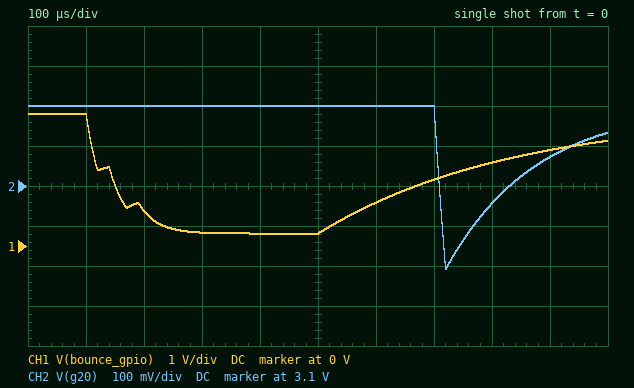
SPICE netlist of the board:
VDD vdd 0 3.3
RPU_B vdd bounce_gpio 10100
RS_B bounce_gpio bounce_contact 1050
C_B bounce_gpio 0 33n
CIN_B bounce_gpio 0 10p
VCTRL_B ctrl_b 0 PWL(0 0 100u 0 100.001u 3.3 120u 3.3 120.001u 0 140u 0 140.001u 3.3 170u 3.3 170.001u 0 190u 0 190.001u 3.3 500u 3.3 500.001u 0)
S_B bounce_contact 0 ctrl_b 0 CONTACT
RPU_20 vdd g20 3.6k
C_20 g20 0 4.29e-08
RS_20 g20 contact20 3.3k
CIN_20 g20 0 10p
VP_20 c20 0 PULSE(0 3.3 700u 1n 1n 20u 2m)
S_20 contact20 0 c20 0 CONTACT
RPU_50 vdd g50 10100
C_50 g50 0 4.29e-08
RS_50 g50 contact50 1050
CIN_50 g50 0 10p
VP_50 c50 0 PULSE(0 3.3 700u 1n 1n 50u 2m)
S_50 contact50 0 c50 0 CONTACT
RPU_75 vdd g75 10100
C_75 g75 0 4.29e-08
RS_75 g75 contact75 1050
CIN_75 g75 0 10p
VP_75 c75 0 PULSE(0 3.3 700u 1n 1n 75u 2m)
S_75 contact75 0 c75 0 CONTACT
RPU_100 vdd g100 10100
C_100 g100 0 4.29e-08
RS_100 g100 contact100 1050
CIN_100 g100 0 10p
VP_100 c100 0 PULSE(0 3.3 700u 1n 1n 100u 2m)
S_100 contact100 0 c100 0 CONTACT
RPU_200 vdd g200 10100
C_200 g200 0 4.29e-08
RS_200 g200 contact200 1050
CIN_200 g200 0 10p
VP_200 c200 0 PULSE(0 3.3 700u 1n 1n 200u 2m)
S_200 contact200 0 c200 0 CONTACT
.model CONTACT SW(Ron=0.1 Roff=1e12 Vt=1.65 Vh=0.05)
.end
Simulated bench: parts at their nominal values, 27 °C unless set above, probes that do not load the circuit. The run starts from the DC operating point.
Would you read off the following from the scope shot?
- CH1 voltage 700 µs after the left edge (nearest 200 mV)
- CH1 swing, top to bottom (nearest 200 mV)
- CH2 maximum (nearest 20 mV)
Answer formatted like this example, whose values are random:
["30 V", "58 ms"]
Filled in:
["1.6 V", "3.0 V", "3.30 V"]
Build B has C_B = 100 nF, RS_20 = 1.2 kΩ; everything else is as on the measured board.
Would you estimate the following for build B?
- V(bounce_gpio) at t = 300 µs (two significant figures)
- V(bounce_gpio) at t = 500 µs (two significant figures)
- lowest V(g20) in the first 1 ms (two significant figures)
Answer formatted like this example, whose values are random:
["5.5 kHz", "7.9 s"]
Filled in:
["880 mV", "380 mV", "2.3 V"]
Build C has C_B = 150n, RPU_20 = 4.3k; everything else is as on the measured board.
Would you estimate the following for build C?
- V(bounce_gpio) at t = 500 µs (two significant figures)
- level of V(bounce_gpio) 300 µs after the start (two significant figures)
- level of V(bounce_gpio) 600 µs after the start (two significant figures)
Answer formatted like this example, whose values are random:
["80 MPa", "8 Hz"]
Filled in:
["550 mV", "1.3 V", "730 mV"]
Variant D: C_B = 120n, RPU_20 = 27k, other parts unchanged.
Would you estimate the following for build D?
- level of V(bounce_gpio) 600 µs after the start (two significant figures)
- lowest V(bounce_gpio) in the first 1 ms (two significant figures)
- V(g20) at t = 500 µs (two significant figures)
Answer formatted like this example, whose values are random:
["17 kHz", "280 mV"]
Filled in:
["670 mV", "440 mV", "3.3 V"]
